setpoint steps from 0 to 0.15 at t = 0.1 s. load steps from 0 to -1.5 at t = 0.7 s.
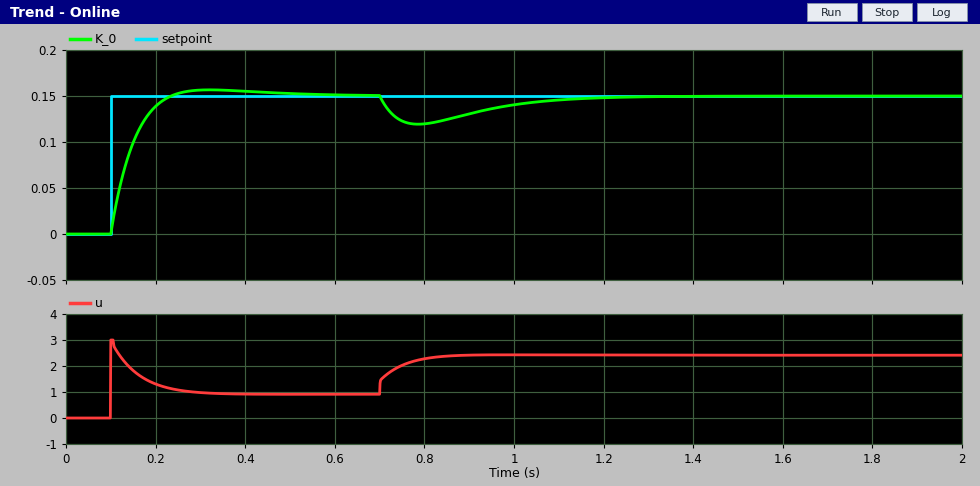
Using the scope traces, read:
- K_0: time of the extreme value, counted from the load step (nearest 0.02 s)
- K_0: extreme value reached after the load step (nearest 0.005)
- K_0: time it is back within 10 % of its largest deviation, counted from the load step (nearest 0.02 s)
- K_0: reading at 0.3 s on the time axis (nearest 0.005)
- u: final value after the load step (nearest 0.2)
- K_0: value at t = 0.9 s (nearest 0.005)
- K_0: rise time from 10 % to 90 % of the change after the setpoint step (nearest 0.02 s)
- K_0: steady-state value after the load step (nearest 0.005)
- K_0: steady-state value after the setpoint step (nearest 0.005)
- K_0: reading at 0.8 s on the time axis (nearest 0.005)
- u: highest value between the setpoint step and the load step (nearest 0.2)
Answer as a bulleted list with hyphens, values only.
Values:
- 0.08 s
- 0.120
- 0.44 s
- 0.155
- 2.4
- 0.130
- 0.08 s
- 0.150
- 0.150
- 0.120
- 3.0
